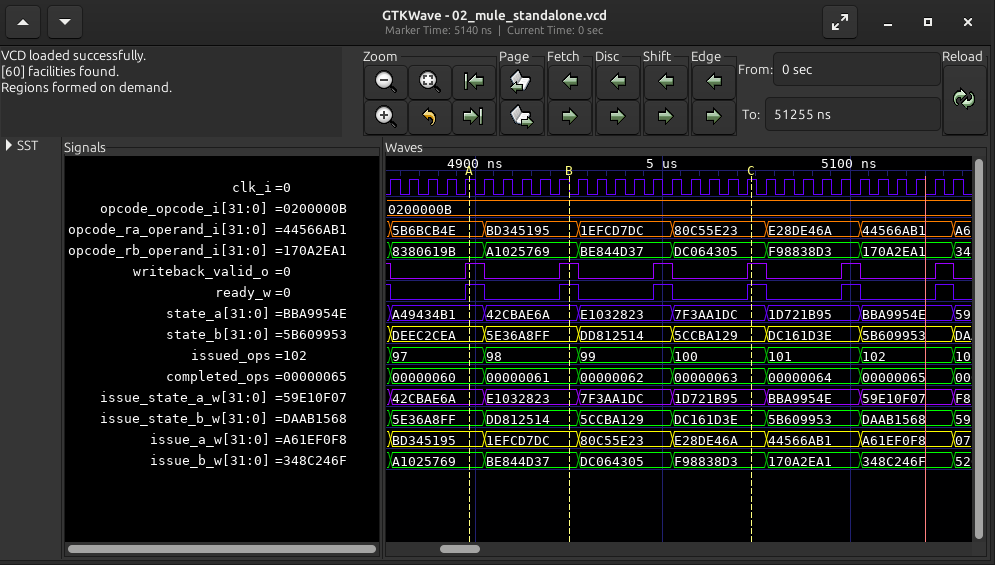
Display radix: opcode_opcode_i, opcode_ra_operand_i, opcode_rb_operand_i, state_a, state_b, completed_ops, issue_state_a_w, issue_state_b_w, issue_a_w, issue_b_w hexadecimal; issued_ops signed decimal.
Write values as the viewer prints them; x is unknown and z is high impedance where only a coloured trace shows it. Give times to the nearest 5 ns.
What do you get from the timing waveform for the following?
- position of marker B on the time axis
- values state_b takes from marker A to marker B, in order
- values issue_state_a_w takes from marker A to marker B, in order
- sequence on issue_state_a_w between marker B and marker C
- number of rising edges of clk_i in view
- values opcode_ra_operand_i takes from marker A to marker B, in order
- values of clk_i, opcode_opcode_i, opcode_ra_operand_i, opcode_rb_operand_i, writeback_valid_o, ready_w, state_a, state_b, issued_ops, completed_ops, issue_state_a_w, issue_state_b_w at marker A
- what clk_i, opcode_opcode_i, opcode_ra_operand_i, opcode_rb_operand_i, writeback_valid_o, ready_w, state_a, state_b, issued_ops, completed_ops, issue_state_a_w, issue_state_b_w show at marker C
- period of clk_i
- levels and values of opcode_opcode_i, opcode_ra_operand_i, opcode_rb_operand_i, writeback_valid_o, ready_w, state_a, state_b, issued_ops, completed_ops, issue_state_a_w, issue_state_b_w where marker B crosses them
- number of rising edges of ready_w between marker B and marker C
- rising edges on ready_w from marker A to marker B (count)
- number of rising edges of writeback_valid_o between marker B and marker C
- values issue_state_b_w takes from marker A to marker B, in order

4950 ns
DEEC2CEA, 5E36A8FF
42CBAE6A, E1032823
E1032823, 7F3AA1DC, 1D721B95
31
5B6BCB4E, BD345195
clk_i=1, opcode_opcode_i=0200000B, opcode_ra_operand_i=5B6BCB4E, opcode_rb_operand_i=8380619B, writeback_valid_o=1, ready_w=1, state_a=A49434B1, state_b=DEEC2CEA, issued_ops=97, completed_ops=00000060, issue_state_a_w=42CBAE6A, issue_state_b_w=5E36A8FF
clk_i=1, opcode_opcode_i=0200000B, opcode_ra_operand_i=80C55E23, opcode_rb_operand_i=DC064305, writeback_valid_o=1, ready_w=1, state_a=7F3AA1DC, state_b=5CCBA129, issued_ops=100, completed_ops=00000063, issue_state_a_w=1D721B95, issue_state_b_w=DC161D3E
10 ns
opcode_opcode_i=0200000B, opcode_ra_operand_i=BD345195, opcode_rb_operand_i=A1025769, writeback_valid_o=1, ready_w=1, state_a=42CBAE6A, state_b=5E36A8FF, issued_ops=98, completed_ops=00000061, issue_state_a_w=E1032823, issue_state_b_w=DD812514
2
1
2
5E36A8FF, DD812514
